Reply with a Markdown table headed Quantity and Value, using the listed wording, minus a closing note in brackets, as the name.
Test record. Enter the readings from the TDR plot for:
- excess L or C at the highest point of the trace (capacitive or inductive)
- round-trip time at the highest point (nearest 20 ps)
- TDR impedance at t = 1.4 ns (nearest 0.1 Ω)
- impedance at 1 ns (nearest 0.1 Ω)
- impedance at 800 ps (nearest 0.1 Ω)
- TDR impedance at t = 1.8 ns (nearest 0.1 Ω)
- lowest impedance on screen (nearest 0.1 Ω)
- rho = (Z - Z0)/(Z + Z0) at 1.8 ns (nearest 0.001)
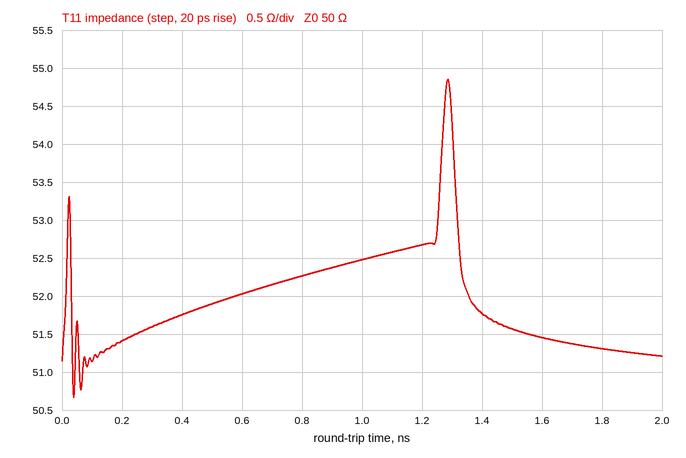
| Quantity | Value |
|---|---|
| excess L or C at the highest point of the trace | inductive |
| round-trip time at the highest point | 1.28 ns |
| TDR impedance at t = 1.4 ns | 51.8 Ω |
| impedance at 1 ns | 52.5 Ω |
| impedance at 800 ps | 52.3 Ω |
| TDR impedance at t = 1.8 ns | 51.3 Ω |
| lowest impedance on screen | 50.7 Ω |
| rho = (Z - Z0)/(Z + Z0) at 1.8 ns | +0.013 |
